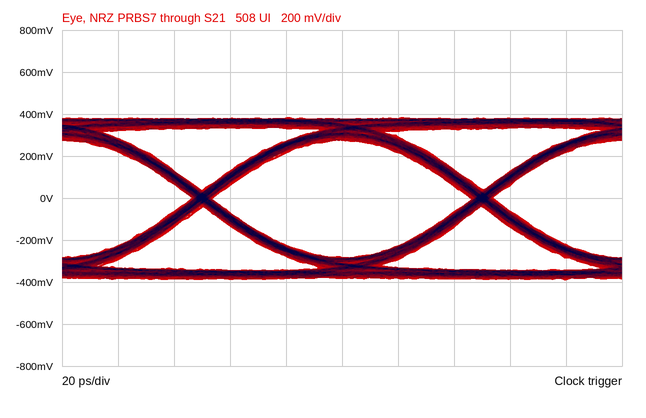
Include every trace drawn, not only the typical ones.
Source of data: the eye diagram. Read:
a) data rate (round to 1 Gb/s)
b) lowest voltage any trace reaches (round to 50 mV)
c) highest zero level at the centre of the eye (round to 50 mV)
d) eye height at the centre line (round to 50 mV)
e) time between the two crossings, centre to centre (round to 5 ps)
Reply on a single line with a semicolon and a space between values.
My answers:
10 Gb/s; -400 mV; -300 mV; 550 mV; 100 ps
